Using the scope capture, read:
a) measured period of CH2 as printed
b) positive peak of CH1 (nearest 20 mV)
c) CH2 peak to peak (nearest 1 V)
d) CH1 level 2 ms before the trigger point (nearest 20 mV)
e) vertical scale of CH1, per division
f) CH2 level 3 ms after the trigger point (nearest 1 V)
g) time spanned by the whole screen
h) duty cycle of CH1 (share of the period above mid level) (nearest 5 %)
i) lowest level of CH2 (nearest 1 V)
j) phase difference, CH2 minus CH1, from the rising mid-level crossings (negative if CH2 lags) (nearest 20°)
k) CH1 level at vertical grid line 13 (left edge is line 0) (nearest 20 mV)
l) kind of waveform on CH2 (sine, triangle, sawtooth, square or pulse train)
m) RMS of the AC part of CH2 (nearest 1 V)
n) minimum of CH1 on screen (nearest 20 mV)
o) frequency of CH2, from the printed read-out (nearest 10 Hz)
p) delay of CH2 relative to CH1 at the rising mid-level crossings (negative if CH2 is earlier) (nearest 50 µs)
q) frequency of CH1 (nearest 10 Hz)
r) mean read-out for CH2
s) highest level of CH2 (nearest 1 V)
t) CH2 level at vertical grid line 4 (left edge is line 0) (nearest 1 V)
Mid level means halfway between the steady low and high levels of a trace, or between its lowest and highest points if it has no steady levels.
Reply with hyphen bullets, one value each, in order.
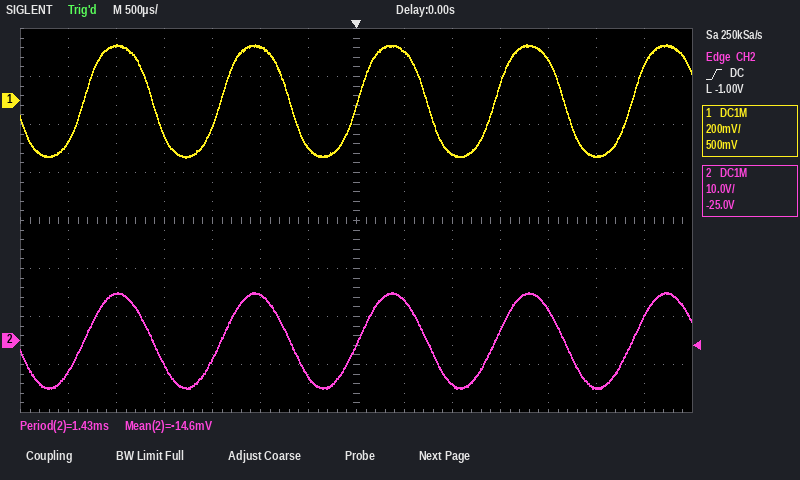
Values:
- 1.43 ms
- 240 mV
- 20 V
- -140 mV
- 200 mV
- 5 V
- 7 ms
- 50 %
- -10 V
- 0°
- 140 mV
- sine
- 7 V
- -240 mV
- 700 Hz
- 0 µs
- 700 Hz
- -14.6 mV
- 10 V
- -4 V
